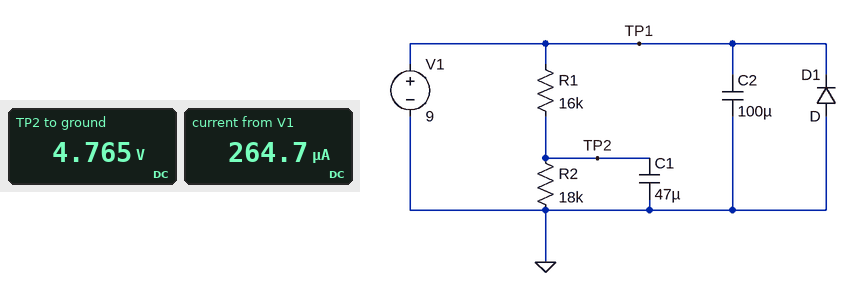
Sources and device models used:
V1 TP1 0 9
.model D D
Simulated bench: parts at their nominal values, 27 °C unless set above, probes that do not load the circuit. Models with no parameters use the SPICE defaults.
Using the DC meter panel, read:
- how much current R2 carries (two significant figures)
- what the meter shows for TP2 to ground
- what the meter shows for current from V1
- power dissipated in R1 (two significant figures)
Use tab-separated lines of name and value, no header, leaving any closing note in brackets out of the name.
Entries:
how much current R2 carries	260 µA
what the meter shows for TP2 to ground	4.765 V
what the meter shows for current from V1	264.7 µA
power dissipated in R1	1.1 mW
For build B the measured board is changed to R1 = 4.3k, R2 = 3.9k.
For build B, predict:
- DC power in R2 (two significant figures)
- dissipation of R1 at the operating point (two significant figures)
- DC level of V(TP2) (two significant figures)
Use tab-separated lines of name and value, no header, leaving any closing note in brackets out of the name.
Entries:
DC power in R2	4.7 mW
dissipation of R1 at the operating point	5.2 mW
DC level of V(TP2)	4.3 V
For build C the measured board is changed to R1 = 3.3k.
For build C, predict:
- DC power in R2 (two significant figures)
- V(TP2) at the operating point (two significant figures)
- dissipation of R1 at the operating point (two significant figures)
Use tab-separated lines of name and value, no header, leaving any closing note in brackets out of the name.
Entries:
DC power in R2	3.2 mW
V(TP2) at the operating point	7.6 V
dissipation of R1 at the operating point	590 µW
